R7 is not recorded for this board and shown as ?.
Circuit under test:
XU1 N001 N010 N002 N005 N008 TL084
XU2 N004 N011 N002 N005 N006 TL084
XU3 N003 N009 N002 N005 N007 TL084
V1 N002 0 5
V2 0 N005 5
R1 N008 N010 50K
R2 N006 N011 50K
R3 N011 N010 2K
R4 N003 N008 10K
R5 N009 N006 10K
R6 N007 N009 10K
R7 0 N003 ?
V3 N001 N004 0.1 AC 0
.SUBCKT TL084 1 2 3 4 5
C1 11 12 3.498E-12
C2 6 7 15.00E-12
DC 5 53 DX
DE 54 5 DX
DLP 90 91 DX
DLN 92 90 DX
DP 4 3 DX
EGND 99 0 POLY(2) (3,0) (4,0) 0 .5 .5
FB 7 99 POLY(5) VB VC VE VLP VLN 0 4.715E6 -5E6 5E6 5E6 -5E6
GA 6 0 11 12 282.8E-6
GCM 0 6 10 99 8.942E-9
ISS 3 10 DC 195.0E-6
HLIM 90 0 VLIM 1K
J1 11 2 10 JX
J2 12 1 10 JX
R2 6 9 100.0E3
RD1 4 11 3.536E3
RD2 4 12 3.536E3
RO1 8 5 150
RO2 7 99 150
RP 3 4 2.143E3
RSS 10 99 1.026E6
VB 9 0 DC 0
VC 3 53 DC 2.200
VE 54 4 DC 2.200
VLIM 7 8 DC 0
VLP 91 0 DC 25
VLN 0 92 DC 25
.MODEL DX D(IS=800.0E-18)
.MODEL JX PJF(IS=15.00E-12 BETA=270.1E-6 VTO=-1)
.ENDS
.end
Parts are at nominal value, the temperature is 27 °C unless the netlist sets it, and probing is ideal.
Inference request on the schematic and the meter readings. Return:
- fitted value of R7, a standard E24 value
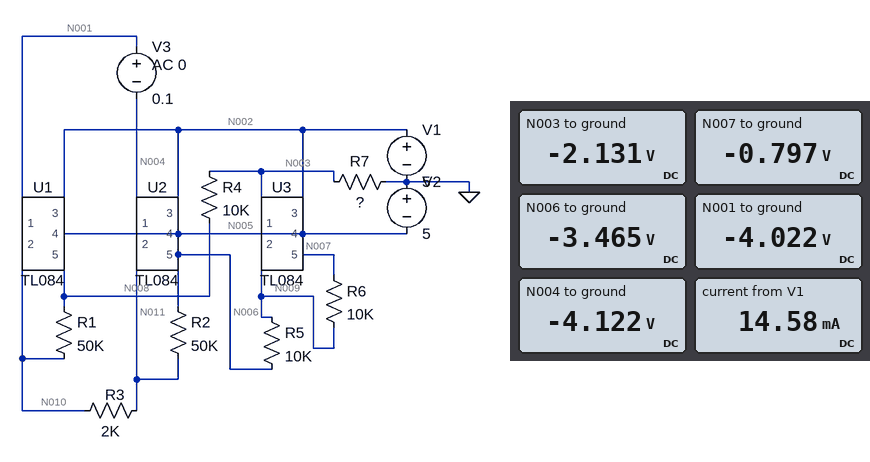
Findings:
16 kΩ
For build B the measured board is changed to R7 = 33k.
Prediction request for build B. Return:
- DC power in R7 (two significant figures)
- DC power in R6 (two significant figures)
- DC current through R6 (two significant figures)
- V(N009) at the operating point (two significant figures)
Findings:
210 µW
65 µW
81 µA
-2.7 V
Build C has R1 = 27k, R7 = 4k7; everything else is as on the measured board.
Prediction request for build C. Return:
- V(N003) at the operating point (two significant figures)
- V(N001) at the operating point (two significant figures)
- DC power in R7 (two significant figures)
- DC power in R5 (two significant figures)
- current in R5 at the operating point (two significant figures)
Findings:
-1.1 V
-4.0 V
260 µW
560 µW
240 µA
